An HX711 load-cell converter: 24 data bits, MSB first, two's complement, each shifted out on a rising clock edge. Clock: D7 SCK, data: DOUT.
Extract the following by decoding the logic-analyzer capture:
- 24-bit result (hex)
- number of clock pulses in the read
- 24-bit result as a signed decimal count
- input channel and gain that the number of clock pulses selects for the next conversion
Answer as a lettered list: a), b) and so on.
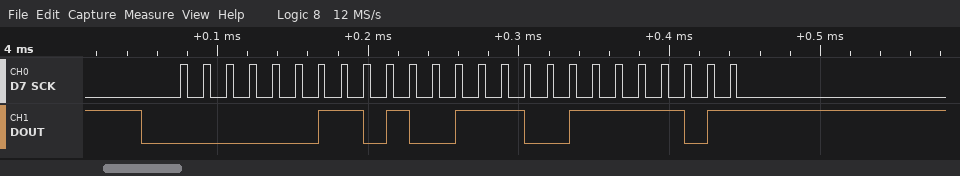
a) 0x034E7D
b) 25
c) 216701
d) channel A, gain 128
